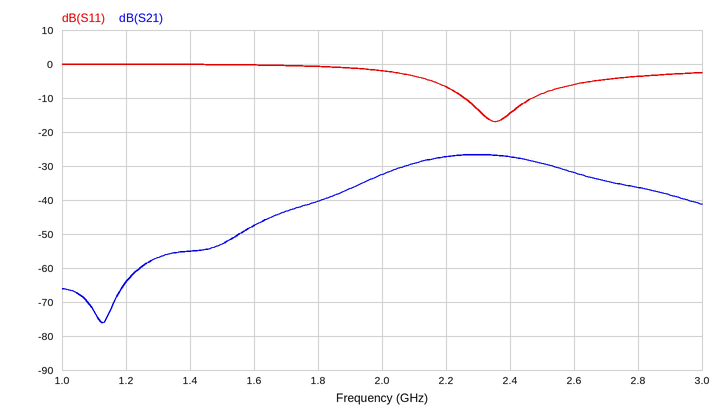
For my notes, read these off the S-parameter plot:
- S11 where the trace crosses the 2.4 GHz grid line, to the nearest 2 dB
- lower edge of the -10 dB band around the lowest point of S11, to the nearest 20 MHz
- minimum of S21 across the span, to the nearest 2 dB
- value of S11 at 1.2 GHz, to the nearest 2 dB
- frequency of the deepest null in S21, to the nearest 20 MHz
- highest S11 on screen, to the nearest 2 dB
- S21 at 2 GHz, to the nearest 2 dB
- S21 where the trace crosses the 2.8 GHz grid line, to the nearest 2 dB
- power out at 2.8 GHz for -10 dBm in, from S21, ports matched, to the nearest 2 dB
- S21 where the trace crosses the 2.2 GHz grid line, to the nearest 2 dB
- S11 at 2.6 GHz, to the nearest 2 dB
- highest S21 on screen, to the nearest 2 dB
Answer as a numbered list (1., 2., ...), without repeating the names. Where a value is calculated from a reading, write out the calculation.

1. -14 dB
2. 2.26 GHz
3. -76 dB
4. 0 dB
5. 1.12 GHz
6. 0 dB
7. -32 dB
8. -36 dB
9. -10 dBm + (-36 dB) = -46 dBm
10. -28 dB
11. -6 dB
12. -26 dB
